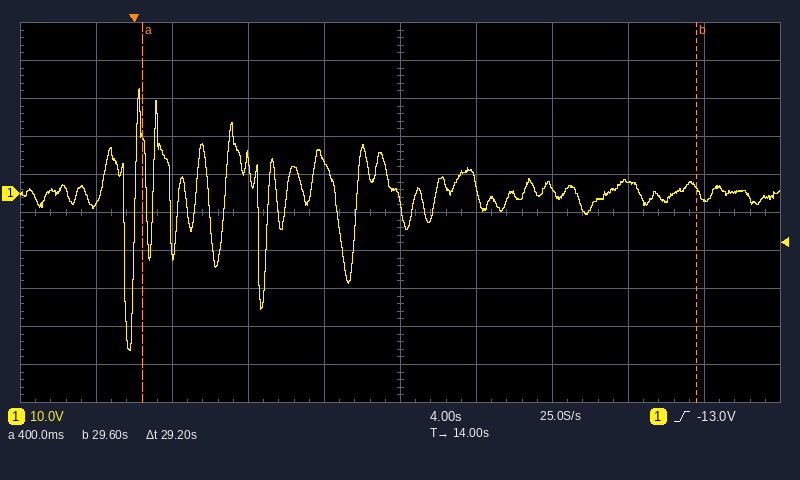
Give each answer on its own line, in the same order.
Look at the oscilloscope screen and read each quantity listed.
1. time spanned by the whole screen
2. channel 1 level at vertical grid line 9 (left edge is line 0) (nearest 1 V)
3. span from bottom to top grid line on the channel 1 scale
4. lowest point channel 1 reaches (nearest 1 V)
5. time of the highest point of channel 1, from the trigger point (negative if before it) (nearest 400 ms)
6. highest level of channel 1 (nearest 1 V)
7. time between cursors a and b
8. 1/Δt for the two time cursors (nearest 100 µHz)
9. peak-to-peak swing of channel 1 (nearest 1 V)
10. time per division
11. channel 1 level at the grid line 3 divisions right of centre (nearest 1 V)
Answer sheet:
40 s
-1 V
100 V
-41 V
+400 ms
28 V
29.2 s
34.2 mHz
69 V
4 s
3 V
